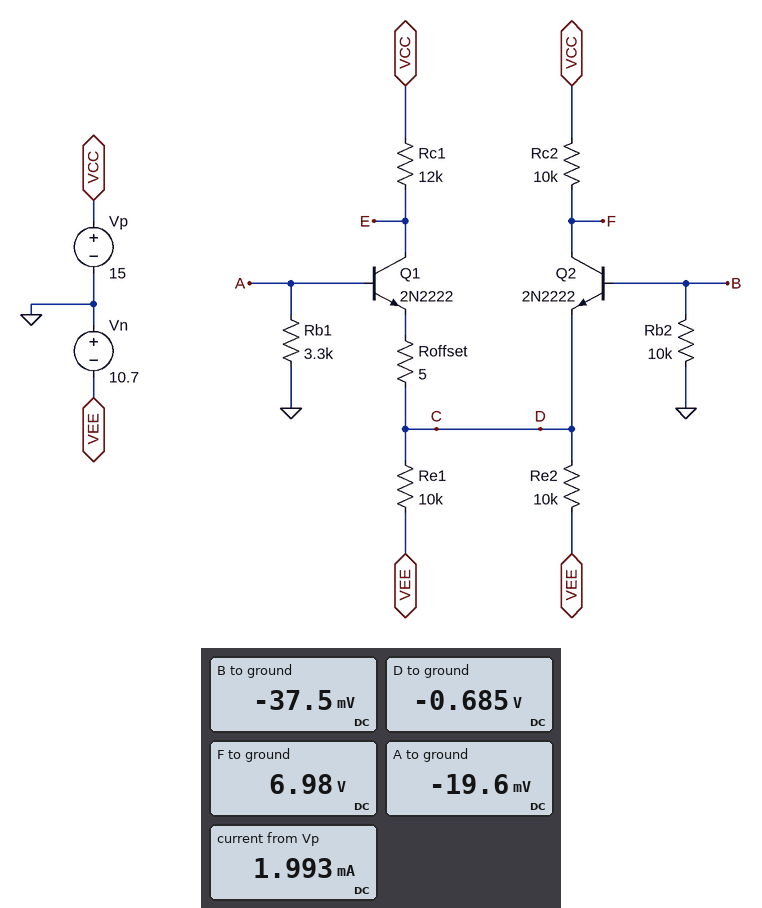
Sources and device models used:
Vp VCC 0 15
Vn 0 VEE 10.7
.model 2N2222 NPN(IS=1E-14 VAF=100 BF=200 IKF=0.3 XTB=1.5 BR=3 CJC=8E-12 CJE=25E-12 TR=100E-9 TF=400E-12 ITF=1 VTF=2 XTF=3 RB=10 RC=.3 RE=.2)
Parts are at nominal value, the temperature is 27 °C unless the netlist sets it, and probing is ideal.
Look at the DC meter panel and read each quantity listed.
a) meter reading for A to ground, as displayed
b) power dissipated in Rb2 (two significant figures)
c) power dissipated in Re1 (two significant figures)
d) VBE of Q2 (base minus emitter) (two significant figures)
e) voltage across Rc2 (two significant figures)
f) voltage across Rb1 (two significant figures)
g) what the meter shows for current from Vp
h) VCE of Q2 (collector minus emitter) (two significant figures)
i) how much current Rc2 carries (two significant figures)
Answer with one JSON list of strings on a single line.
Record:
["-19.6 mV", "140 nW", "10 mW", "650 mV", "8.0 V", "20 mV", "1.993 mA", "7.7 V", "800 µA"]
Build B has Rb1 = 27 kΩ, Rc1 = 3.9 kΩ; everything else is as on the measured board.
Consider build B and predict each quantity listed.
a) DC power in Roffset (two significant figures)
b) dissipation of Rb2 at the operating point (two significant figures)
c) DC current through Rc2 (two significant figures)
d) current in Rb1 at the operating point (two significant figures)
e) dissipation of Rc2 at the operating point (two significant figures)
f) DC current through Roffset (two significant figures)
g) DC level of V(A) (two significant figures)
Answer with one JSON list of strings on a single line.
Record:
["2.3 µW", "420 nW", "1.3 mA", "3.0 µA", "17 mW", "680 µA", "-81 mV"]
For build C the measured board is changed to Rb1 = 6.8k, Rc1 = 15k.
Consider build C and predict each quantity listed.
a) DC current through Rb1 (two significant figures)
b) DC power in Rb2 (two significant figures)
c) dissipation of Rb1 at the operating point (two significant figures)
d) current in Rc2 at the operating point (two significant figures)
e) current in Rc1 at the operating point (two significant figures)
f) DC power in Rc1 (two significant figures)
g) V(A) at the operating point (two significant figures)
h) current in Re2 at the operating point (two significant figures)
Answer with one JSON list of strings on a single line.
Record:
["5.4 µA", "210 nW", "200 nW", "960 µA", "1.0 mA", "16 mW", "-37 mV", "1.0 mA"]
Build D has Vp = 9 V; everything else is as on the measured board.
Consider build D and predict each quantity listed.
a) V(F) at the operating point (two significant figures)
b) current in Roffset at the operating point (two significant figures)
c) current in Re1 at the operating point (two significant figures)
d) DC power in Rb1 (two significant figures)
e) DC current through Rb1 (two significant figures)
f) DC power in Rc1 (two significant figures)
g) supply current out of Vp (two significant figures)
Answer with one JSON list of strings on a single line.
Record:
["-910 mV", "920 µA", "970 µA", "29 µW", "94 µA", "8.2 mW", "1.8 mA"]
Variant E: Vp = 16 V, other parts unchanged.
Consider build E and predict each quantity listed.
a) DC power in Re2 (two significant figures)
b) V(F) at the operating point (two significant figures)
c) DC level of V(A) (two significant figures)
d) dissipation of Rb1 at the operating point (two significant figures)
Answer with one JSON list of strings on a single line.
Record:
["10 mW", "8.0 V", "-19 mV", "110 nW"]
